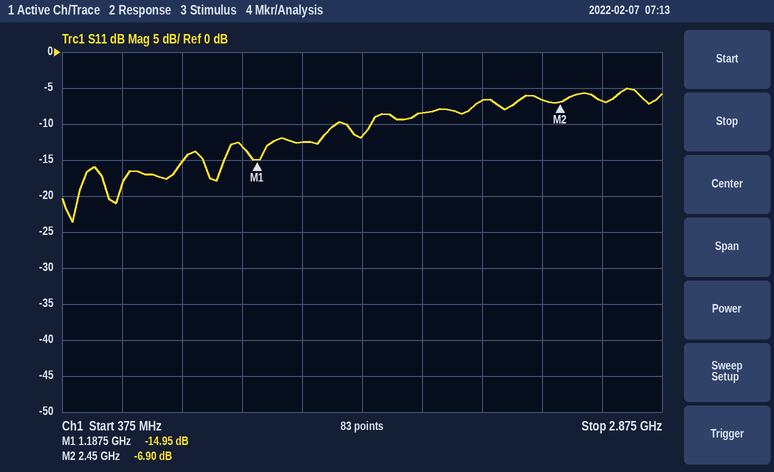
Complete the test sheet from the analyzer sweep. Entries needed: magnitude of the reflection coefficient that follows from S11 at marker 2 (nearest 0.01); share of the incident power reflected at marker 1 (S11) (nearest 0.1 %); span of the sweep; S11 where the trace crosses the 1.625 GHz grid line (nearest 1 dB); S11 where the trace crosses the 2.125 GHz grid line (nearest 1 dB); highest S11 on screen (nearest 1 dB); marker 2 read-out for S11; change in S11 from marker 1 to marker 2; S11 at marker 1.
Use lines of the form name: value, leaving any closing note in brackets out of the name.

magnitude of the reflection coefficient that follows from S11 at marker 2: 0.45
share of the incident power reflected at marker 1 (S11): 3.2 %
span of the sweep: 2.5 GHz
S11 where the trace crosses the 1.625 GHz grid line: -12 dB
S11 where the trace crosses the 2.125 GHz grid line: -7 dB
highest S11 on screen: -5 dB
marker 2 read-out for S11: -6.90 dB
change in S11 from marker 1 to marker 2: 8.05 dB
S11 at marker 1: -14.95 dB
